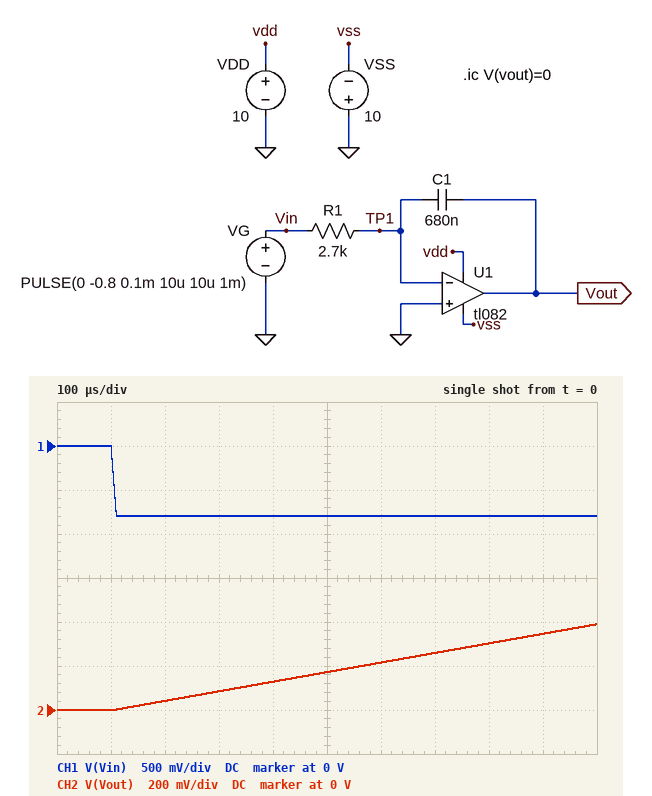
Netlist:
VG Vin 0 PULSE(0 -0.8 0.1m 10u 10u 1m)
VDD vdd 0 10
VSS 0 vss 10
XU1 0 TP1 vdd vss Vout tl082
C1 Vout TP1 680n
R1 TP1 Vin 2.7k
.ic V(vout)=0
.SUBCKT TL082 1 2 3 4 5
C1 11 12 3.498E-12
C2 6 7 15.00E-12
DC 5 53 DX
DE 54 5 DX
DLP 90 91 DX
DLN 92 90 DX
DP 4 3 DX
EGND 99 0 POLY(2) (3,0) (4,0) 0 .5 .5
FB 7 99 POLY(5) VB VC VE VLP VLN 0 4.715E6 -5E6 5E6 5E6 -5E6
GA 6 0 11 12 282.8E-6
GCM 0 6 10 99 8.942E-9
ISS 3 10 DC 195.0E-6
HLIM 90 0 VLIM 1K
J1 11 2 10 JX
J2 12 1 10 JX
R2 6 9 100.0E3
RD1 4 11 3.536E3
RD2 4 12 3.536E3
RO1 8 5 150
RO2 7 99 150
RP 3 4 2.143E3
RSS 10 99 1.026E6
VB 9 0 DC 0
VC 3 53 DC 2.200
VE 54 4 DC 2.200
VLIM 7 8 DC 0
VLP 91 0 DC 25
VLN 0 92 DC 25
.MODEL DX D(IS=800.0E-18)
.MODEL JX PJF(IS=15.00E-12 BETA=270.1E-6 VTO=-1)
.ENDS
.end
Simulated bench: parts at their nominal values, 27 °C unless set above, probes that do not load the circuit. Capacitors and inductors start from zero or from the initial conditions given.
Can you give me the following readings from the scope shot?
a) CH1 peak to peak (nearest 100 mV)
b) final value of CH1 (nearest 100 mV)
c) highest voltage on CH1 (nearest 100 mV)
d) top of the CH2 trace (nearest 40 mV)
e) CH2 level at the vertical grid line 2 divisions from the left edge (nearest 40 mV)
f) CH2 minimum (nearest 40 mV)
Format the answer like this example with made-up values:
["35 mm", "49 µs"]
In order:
["800 mV", "-800 mV", "0 V", "400 mV", "40 mV", "0 V"]
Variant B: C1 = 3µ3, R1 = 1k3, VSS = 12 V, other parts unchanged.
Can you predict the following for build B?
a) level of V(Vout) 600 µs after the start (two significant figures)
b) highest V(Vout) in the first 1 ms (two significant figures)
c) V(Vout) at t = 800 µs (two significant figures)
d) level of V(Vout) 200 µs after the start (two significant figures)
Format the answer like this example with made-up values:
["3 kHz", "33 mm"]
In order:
["92 mV", "170 mV", "130 mV", "18 mV"]
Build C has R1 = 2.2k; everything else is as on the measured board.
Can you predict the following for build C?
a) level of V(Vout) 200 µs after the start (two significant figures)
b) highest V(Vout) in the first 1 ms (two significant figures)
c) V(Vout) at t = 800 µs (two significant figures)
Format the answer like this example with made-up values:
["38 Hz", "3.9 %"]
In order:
["51 mV", "480 mV", "370 mV"]
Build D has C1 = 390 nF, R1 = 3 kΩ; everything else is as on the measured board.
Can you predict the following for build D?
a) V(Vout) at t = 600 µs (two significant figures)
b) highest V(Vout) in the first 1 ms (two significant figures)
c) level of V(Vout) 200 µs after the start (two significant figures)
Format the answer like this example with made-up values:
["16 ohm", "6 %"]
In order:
["340 mV", "610 mV", "65 mV"]
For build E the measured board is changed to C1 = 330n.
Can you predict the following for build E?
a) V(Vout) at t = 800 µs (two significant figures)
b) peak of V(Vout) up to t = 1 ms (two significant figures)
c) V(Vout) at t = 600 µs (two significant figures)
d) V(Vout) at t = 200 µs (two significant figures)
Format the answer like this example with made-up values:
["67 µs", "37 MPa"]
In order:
["620 mV", "800 mV", "440 mV", "85 mV"]
